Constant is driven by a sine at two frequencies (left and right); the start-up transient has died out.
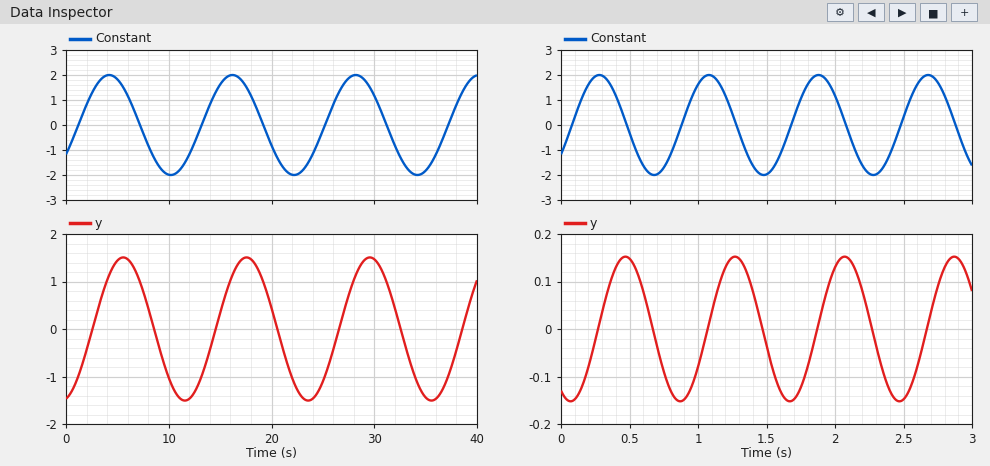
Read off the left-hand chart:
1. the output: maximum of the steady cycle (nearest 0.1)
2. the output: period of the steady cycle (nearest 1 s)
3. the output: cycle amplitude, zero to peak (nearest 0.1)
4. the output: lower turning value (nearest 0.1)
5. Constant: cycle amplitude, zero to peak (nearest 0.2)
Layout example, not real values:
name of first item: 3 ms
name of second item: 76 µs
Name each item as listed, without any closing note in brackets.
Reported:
the output: maximum of the steady cycle: 1.5
the output: period of the steady cycle: 12 s
the output: cycle amplitude, zero to peak: 1.5
the output: lower turning value: -1.5
Constant: cycle amplitude, zero to peak: 2.0
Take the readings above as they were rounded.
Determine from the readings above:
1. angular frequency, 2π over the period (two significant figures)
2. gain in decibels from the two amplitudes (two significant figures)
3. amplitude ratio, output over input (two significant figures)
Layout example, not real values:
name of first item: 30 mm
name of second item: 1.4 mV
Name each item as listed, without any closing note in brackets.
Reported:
angular frequency, 2π over the period: 0.52 rad/s
gain in decibels from the two amplitudes: -2.5 dB
amplitude ratio, output over input: 0.75
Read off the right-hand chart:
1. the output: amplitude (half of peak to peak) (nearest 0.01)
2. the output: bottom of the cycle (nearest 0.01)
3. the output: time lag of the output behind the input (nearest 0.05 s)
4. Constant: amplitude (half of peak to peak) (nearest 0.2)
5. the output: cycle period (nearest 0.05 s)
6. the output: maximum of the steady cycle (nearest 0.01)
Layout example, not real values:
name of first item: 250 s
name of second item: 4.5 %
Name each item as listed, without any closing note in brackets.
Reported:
the output: amplitude (half of peak to peak): 0.15
the output: bottom of the cycle: -0.15
the output: time lag of the output behind the input: 0.20 s
Constant: amplitude (half of peak to peak): 2.0
the output: cycle period: 0.80 s
the output: maximum of the steady cycle: 0.15
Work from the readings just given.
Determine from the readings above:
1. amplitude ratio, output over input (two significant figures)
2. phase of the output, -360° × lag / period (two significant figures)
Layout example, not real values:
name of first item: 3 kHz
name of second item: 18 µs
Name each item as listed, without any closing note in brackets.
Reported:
amplitude ratio, output over input: 0.075
phase of the output, -360° × lag / period: -90°
